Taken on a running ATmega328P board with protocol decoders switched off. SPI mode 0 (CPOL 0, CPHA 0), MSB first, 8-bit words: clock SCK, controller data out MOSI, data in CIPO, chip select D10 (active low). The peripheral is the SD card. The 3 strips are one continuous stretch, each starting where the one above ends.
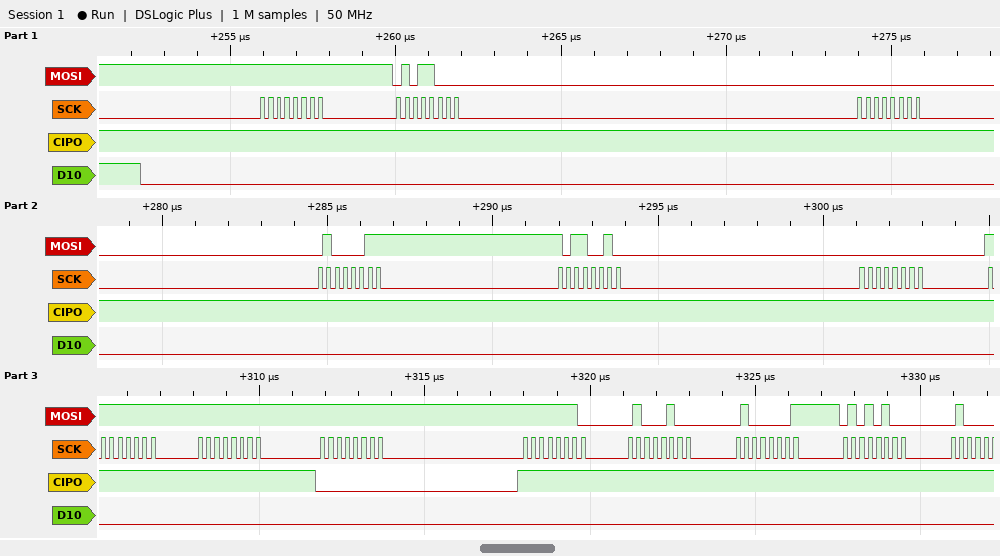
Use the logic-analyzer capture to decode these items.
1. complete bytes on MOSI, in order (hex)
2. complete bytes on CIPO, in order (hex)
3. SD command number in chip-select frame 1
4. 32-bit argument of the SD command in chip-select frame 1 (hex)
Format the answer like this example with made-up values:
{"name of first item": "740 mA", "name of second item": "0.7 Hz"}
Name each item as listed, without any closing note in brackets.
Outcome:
{"complete bytes on MOSI, in order": "0xFF 0x58 0x00 0x43 0xB2 0x00 0xFF 0xFF 0xFF 0xFE 0x44 0x41 0x54", "complete bytes on CIPO, in order": "0xFF 0xFF 0xFF 0xFF 0xFF 0xFF 0xFF 0xFF 0x00 0xFF 0xFF 0xFF 0xFF", "SD command number in chip-select frame 1": "CMD24", "32-bit argument of the SD command in chip-select frame 1": "0x0043B200"}
